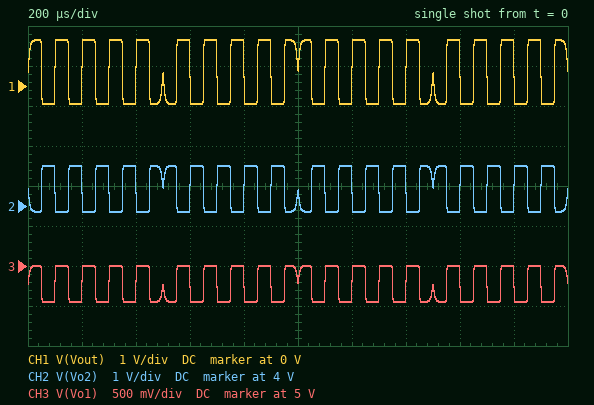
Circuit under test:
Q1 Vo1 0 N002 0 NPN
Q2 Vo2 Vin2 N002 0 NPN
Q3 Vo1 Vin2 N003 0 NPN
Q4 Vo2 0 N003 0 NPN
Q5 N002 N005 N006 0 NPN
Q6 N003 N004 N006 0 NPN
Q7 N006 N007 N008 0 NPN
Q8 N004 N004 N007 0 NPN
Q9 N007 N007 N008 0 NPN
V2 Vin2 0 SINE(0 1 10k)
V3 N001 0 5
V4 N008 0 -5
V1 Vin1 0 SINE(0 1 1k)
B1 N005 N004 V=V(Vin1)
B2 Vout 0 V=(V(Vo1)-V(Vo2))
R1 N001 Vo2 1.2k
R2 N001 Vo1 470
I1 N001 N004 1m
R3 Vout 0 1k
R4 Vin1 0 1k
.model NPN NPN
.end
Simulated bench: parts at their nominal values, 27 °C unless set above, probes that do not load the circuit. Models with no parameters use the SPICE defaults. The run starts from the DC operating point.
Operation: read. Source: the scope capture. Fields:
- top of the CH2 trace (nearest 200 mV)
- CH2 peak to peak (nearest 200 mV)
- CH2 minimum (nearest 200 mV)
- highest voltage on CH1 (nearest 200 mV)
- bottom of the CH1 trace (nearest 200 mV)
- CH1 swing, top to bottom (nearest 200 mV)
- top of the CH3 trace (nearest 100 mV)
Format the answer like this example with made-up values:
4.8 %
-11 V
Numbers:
5.0 V
1.2 V
3.8 V
1.2 V
-400 mV
1.6 V
5.0 V
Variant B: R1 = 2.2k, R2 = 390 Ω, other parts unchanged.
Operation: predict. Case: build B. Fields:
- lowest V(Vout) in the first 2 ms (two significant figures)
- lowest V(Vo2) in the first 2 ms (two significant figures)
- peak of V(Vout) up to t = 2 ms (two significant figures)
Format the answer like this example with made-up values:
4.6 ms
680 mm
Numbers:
-370 mV
2.9 V
2.1 V
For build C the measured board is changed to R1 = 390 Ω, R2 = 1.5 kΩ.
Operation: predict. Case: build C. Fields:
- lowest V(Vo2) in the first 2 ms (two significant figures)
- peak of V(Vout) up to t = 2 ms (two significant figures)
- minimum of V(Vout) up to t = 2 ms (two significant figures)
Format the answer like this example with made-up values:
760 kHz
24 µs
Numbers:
4.6 V
370 mV
-1.4 V
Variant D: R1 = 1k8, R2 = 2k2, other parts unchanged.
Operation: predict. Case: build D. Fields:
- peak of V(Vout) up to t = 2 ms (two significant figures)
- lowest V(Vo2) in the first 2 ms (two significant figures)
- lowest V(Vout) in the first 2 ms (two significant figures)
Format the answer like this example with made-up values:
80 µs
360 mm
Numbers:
1.7 V
3.3 V
-2.1 V
